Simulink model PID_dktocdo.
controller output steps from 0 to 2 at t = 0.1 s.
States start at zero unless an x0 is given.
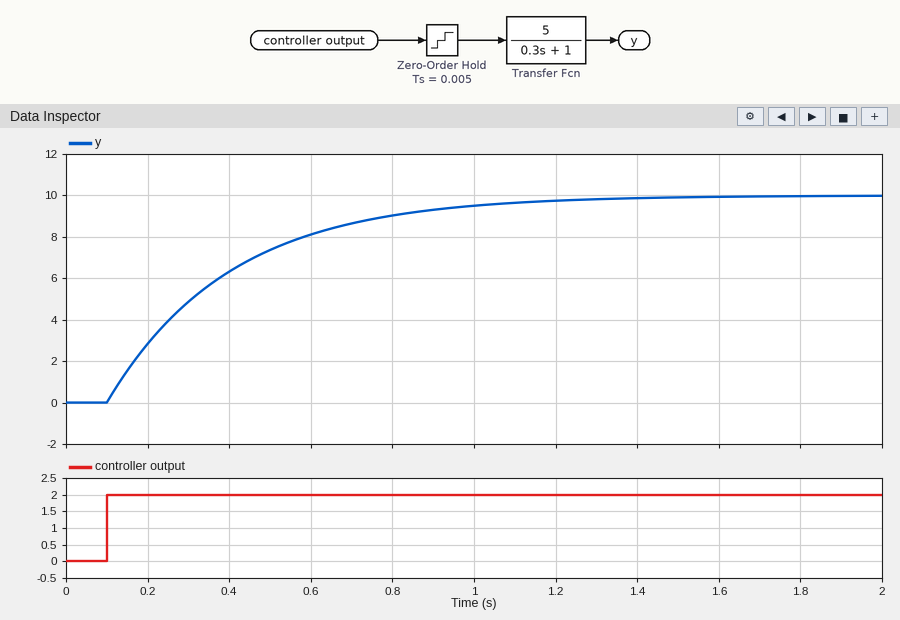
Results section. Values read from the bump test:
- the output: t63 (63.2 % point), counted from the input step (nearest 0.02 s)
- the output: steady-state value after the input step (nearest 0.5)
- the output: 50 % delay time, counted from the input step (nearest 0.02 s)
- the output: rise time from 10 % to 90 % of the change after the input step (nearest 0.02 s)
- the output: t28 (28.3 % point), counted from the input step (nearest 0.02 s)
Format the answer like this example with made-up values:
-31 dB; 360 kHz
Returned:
0.30 s; 10.0; 0.20 s; 0.66 s; 0.10 s
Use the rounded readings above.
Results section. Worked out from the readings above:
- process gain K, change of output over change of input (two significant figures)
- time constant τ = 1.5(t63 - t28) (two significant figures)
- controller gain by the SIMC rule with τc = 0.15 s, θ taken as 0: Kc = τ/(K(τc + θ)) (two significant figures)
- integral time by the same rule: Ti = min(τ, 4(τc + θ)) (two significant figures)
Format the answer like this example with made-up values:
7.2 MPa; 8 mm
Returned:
5.0; 0.30 s; 0.40; 0.30 s
